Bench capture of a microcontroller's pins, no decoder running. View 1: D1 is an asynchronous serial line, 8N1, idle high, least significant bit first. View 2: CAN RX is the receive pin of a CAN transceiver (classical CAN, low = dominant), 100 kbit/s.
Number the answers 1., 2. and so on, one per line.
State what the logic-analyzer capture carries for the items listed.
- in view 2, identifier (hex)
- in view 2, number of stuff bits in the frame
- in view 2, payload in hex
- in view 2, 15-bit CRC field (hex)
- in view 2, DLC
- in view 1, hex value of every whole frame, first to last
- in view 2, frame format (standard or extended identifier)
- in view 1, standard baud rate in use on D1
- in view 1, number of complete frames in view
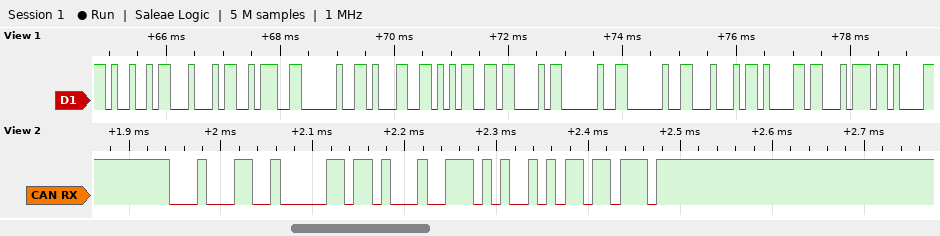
1. 0x119
2. 1
3. D1 3A
4. 0x4ADB
5. 2
6. 0x49 0x44 0x3A 0x20 0x31 0x35 0x43 0x20 0x20 0x44 0x61 0x74
7. standard
8. 9600 baud
9. 12
